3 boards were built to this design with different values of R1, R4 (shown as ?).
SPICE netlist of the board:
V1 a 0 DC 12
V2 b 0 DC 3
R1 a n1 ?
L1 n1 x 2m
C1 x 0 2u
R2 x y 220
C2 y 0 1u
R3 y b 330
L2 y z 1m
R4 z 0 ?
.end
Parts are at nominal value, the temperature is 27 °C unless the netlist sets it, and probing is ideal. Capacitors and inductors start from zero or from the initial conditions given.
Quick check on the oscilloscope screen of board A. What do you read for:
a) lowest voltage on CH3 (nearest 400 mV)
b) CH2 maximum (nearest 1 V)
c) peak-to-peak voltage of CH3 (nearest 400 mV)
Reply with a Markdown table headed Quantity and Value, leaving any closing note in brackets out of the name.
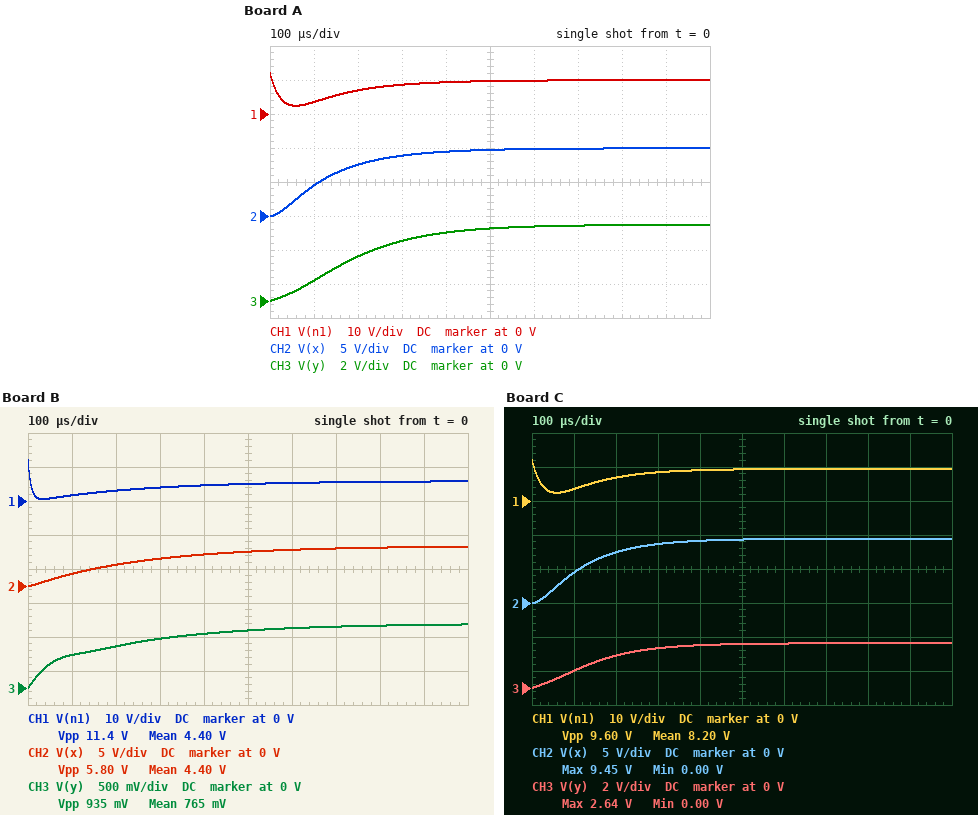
| Quantity | Value |
|---|---|
| lowest voltage on CH3 | 0 V |
| CH2 maximum | 10 V |
| peak-to-peak voltage of CH3 | 4.4 V |
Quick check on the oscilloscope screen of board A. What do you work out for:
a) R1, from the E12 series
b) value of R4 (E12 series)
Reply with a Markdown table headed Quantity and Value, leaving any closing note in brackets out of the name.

| Quantity | Value |
|---|---|
| R1, from the E12 series | 82 Ω |
| value of R4 | 220 Ω |
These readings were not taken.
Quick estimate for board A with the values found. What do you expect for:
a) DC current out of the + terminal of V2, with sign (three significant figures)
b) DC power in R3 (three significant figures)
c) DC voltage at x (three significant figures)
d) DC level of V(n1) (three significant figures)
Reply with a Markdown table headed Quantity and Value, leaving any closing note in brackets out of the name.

| Quantity | Value |
|---|---|
| DC current out of the + terminal of V2, with sign | -4.50 mA |
| DC power in R3 | 6.68 mW |
| DC voltage at x | 9.96 V |
| DC level of V(n1) | 9.96 V |
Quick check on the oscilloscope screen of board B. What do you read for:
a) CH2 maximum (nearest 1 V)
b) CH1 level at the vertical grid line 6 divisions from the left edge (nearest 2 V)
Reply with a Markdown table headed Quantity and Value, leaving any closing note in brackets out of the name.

| Quantity | Value |
|---|---|
| CH2 maximum | 6 V |
| CH1 level at the vertical grid line 6 divisions from the left edge | 6 V |
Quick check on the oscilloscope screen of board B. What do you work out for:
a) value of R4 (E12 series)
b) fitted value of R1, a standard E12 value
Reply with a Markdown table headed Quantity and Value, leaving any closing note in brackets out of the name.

| Quantity | Value |
|---|---|
| value of R4 | 33 Ω |
| fitted value of R1, a standard E12 value | 270 Ω |
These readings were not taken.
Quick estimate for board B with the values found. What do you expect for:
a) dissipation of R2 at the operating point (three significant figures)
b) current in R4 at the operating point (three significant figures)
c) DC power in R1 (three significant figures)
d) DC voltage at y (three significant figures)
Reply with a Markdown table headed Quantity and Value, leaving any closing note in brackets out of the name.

| Quantity | Value |
|---|---|
| dissipation of R2 at the operating point | 112 mW |
| current in R4 at the operating point | 28.8 mA |
| DC power in R1 | 137 mW |
| DC voltage at y | 949 mV |
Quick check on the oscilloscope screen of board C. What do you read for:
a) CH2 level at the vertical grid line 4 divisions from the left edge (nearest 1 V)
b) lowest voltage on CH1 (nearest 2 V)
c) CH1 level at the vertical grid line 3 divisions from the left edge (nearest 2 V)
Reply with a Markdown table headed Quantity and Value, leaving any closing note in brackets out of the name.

| Quantity | Value |
|---|---|
| CH2 level at the vertical grid line 4 divisions from the left edge | 9 V |
| lowest voltage on CH1 | 2 V |
| CH1 level at the vertical grid line 3 divisions from the left edge | 8 V |
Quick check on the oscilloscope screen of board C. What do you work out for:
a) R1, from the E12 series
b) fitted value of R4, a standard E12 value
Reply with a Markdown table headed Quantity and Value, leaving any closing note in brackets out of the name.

| Quantity | Value |
|---|---|
| R1, from the E12 series | 82 Ω |
| fitted value of R4, a standard E12 value | 82 Ω |
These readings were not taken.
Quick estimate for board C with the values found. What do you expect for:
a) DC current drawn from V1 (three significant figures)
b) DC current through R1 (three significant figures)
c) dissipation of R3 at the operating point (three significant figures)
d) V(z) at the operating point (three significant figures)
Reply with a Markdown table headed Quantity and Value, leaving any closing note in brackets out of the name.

| Quantity | Value |
|---|---|
| DC current drawn from V1 | 31.0 mA |
| DC current through R1 | 31.0 mA |
| dissipation of R3 at the operating point | 406 µW |
| V(z) at the operating point | 2.63 V |
